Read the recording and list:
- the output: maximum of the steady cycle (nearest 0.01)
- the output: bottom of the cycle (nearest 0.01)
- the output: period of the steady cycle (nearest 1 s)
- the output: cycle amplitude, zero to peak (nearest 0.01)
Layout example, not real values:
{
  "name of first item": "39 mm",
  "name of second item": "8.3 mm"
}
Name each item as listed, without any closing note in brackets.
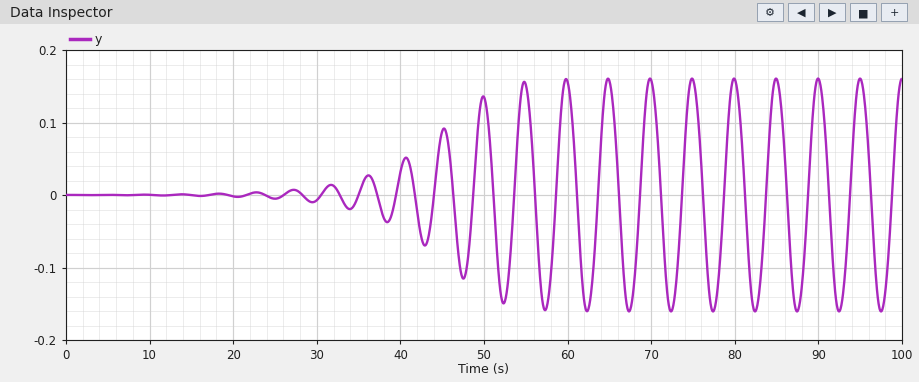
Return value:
{
  "the output: maximum of the steady cycle": "0.16",
  "the output: bottom of the cycle": "-0.16",
  "the output: period of the steady cycle": "5 s",
  "the output: cycle amplitude, zero to peak": "0.16"
}
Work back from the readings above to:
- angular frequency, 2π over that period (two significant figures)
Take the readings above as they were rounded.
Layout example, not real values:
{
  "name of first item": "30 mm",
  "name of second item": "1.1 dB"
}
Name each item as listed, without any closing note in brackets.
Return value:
{
  "angular frequency, 2π over that period": "1.3 rad/s"
}
